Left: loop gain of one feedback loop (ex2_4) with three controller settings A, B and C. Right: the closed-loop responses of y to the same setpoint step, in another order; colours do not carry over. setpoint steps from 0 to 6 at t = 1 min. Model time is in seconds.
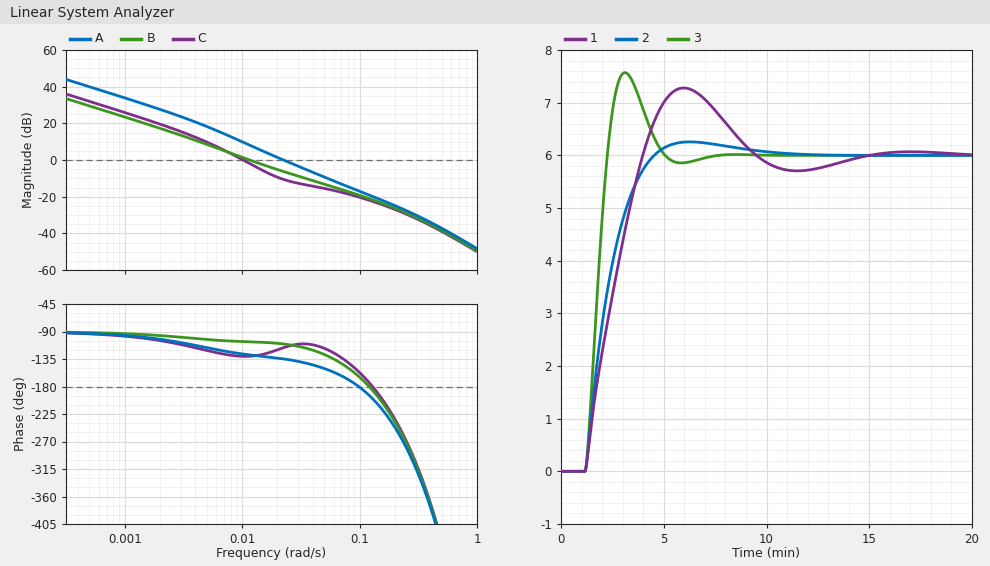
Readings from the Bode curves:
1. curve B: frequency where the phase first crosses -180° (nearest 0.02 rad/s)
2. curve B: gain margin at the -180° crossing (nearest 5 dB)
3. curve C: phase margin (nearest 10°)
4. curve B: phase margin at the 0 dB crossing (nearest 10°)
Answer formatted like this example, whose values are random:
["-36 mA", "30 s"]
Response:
["0.12 rad/s", "20 dB", "50°", "70°"]
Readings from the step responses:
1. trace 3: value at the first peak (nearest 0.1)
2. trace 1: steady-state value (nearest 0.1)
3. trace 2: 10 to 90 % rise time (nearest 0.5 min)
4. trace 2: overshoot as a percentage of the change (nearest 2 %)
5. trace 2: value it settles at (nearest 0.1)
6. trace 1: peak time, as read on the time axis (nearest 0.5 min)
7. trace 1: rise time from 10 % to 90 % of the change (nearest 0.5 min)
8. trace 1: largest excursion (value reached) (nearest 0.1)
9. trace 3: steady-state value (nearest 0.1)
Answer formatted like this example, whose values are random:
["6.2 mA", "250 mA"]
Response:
["7.6", "6.0", "2.0 min", "4 %", "6.0", "6.0 min", "2.0 min", "7.3", "6.0"]
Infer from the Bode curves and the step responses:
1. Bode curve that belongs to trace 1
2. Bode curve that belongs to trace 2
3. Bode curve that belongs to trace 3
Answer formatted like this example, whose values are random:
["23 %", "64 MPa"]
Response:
["C", "B", "A"]
